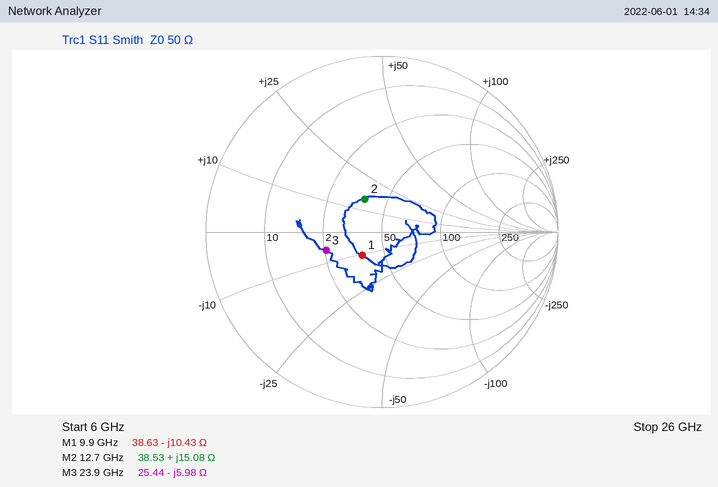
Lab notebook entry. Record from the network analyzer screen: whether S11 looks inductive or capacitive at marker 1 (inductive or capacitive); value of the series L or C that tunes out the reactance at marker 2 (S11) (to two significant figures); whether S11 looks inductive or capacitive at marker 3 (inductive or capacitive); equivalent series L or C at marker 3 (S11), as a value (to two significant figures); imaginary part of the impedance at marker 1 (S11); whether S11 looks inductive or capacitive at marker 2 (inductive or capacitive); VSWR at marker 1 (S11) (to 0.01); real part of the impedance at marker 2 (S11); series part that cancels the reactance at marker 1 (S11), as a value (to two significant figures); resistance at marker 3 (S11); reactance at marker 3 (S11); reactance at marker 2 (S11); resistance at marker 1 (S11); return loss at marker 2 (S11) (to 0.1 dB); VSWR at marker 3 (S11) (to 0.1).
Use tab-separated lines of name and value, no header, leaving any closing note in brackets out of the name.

whether S11 looks inductive or capacitive at marker 1	capacitive
value of the series L or C that tunes out the reactance at marker 2 (S11)	830 fF
whether S11 looks inductive or capacitive at marker 3	capacitive
equivalent series L or C at marker 3 (S11), as a value	1.1 pF
imaginary part of the impedance at marker 1	-10.43 Ω
whether S11 looks inductive or capacitive at marker 2	inductive
VSWR at marker 1 (S11)	1.42
real part of the impedance at marker 2	38.53 Ω
series part that cancels the reactance at marker 1 (S11), as a value	170 pH
resistance at marker 3	25.44 Ω
reactance at marker 3	-5.98 Ω
reactance at marker 2	+15.08 Ω
resistance at marker 1	38.63 Ω
return loss at marker 2 (S11)	13.5 dB
VSWR at marker 3 (S11)	2.0
